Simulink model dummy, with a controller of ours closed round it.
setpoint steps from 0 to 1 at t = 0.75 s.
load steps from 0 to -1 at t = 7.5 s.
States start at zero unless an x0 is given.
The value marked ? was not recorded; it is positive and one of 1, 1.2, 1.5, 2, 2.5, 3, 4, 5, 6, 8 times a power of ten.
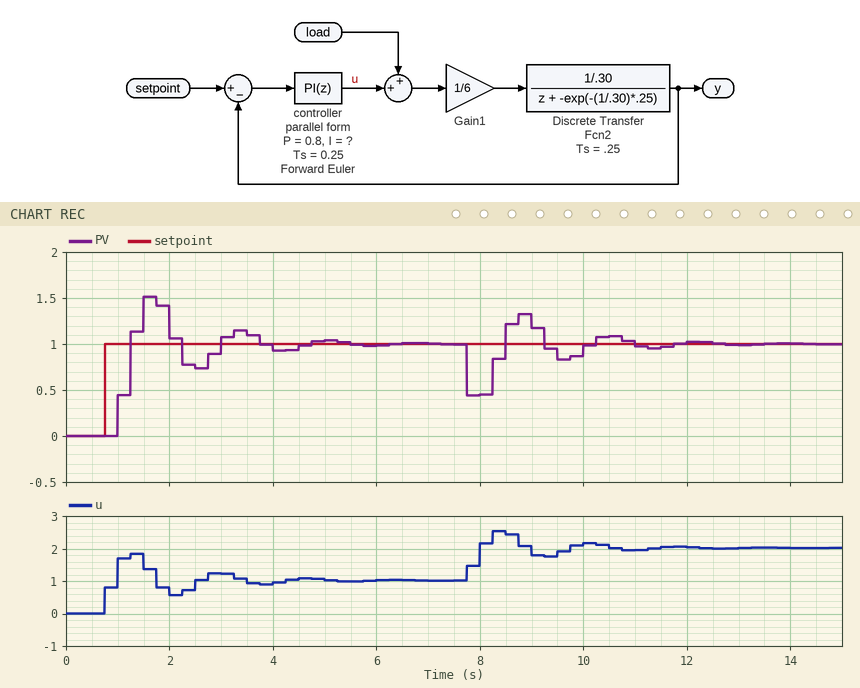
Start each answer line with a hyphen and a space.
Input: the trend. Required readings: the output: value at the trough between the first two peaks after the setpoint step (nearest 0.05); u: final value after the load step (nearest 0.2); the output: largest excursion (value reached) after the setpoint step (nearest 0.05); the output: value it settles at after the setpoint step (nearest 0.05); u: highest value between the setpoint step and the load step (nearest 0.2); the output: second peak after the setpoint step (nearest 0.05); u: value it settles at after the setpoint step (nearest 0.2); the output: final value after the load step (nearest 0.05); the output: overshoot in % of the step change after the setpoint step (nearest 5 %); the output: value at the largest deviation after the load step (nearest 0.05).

- 0.75
- 2.0
- 1.50
- 1.00
- 1.8
- 1.15
- 1.0
- 1.00
- 50 %
- 0.45
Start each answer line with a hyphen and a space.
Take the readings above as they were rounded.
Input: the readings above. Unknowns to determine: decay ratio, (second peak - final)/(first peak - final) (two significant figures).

- 0.30
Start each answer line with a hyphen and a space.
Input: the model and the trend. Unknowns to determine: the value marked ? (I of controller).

- 5
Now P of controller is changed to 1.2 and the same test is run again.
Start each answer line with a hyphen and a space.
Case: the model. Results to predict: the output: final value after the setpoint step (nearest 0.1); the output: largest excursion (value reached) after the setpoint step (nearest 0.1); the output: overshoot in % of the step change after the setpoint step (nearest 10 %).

- 1.0
- 1.3
- 30 %
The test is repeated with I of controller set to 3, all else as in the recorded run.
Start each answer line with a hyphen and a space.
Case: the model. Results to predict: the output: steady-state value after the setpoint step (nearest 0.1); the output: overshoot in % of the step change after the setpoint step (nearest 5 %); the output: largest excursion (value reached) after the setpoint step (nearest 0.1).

- 1.0
- 15 %
- 1.1
